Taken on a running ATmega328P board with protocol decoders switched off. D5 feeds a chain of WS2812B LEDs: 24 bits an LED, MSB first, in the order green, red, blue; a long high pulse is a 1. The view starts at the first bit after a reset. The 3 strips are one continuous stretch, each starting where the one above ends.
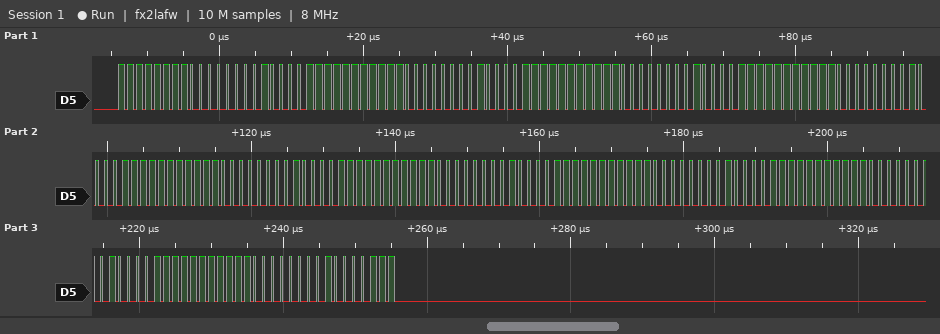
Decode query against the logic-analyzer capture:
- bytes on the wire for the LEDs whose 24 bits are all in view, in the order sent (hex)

FF 00 87 FF 00 87 FF 00 87 FF 00 87 FF 00 87 FF 00 87 FF 00 87 FF 00 87 FF 00 87
